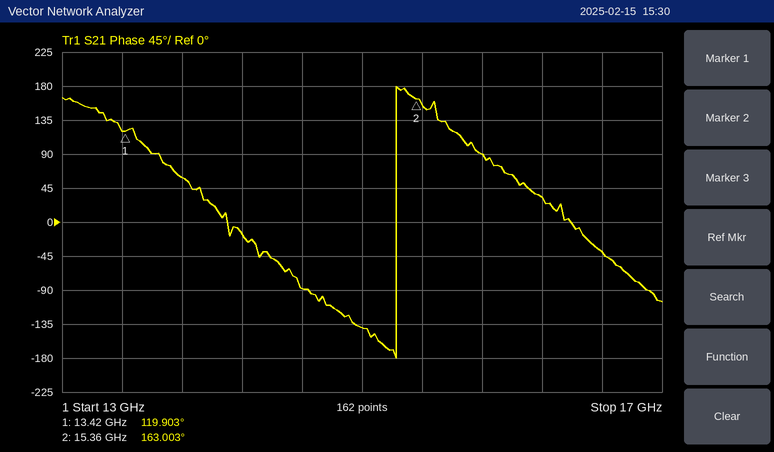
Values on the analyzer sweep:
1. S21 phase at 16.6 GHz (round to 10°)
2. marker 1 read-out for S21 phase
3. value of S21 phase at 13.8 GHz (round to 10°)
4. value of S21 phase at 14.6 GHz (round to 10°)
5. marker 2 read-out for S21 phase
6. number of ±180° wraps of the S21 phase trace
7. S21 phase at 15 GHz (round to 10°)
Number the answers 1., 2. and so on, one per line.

1. -40°
2. 119.903°
3. 60°
4. -90°
5. 163.003°
6. 1
7. -140°
